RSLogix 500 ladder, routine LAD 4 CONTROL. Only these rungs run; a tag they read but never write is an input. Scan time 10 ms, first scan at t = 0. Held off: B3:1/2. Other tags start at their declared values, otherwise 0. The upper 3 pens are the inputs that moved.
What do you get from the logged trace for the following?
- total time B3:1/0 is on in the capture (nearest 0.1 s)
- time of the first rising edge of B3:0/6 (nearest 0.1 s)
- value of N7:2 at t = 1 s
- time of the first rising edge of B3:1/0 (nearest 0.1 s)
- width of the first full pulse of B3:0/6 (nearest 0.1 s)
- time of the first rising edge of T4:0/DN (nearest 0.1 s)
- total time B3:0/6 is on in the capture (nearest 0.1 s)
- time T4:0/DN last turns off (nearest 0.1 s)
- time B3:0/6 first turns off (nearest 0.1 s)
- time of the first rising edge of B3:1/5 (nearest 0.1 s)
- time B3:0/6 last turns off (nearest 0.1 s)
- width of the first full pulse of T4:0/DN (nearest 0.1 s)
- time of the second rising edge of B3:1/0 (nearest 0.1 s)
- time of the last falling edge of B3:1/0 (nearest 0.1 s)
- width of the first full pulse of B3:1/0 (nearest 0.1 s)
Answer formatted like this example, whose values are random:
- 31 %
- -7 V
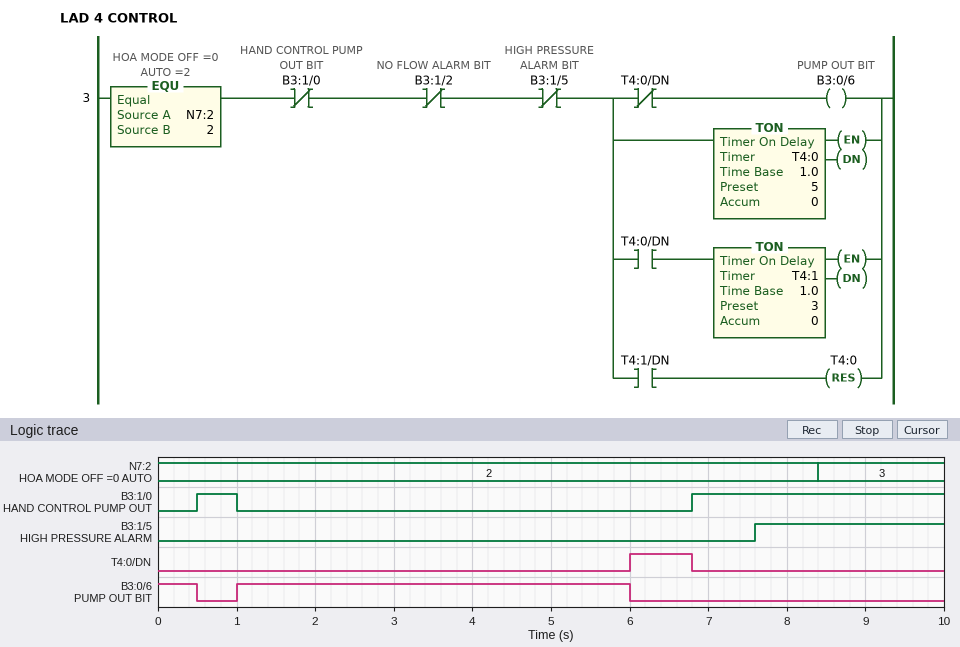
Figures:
- 3.7 s
- 1.0 s
- 2
- 0.5 s
- 5.0 s
- 6.0 s
- 5.5 s
- 6.8 s
- 0.5 s
- 7.6 s
- 6.0 s
- 0.8 s
- 6.8 s
- 1.0 s
- 0.5 s
